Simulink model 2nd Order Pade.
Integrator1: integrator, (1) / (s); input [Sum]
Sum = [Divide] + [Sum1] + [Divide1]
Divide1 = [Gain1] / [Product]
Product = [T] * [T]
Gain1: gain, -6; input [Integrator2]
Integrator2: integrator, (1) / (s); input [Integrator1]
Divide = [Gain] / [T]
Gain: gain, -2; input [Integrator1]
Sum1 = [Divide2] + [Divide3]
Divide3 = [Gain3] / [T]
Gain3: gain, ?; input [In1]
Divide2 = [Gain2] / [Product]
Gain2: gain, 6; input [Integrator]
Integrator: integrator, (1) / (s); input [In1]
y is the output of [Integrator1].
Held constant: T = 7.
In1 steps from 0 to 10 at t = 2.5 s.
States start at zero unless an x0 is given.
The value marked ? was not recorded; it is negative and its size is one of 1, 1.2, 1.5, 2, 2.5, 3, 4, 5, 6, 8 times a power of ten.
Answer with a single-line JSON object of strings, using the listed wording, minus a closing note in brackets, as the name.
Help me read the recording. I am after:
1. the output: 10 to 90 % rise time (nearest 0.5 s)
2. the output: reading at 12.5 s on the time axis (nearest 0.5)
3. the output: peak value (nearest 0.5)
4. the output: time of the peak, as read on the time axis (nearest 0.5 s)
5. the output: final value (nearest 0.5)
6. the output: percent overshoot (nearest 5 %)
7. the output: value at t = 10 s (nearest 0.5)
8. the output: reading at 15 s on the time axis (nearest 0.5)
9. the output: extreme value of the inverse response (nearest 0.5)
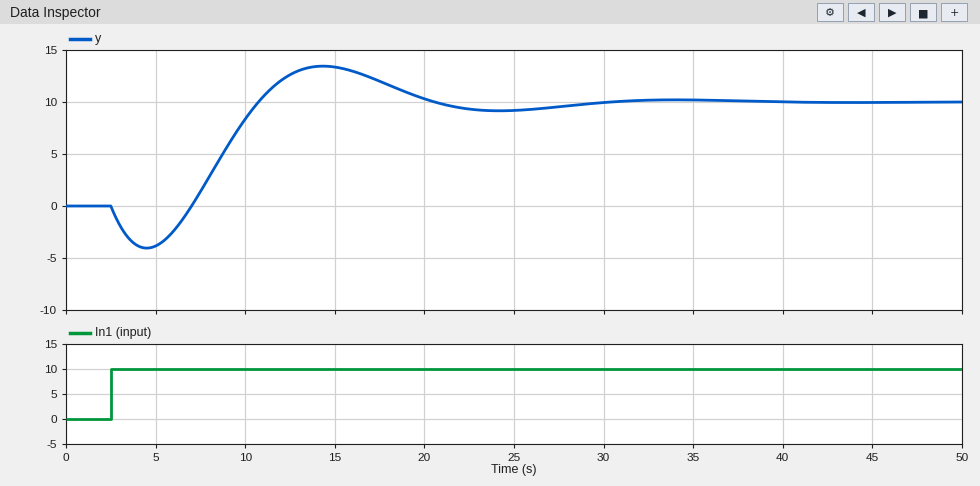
{"the output: 10 to 90 % rise time": "3.0 s", "the output: reading at 12.5 s on the time axis": "12.5", "the output: peak value": "13.5", "the output: time of the peak, as read on the time axis": "14.5 s", "the output: final value": "10.0", "the output: percent overshoot": "35 %", "the output: value at t = 10 s": "8.5", "the output: reading at 15 s on the time axis": "13.5", "the output: extreme value of the inverse response": "-4.0"}
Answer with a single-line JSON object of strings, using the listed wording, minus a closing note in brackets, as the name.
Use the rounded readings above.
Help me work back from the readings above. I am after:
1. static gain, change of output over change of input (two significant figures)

{"static gain, change of output over change of input": "1.0"}
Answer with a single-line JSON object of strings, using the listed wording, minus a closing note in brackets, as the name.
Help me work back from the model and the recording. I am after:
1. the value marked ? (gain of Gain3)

{"the value marked ?": "-3"}
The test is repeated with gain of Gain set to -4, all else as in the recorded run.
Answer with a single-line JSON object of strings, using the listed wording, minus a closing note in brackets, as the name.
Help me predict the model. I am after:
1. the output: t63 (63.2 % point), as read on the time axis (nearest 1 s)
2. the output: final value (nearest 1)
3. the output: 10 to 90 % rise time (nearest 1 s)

{"the output: t63 (63.2 % point), as read on the time axis": "10 s", "the output: final value": "10", "the output: 10 to 90 % rise time": "6 s"}
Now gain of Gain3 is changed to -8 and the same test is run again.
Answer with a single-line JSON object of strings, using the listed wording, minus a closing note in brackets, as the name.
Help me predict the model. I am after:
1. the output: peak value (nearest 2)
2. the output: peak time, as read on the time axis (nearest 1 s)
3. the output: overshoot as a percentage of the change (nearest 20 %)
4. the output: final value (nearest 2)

{"the output: peak value": "16", "the output: peak time, as read on the time axis": "15 s", "the output: overshoot as a percentage of the change": "60 %", "the output: final value": "10"}
